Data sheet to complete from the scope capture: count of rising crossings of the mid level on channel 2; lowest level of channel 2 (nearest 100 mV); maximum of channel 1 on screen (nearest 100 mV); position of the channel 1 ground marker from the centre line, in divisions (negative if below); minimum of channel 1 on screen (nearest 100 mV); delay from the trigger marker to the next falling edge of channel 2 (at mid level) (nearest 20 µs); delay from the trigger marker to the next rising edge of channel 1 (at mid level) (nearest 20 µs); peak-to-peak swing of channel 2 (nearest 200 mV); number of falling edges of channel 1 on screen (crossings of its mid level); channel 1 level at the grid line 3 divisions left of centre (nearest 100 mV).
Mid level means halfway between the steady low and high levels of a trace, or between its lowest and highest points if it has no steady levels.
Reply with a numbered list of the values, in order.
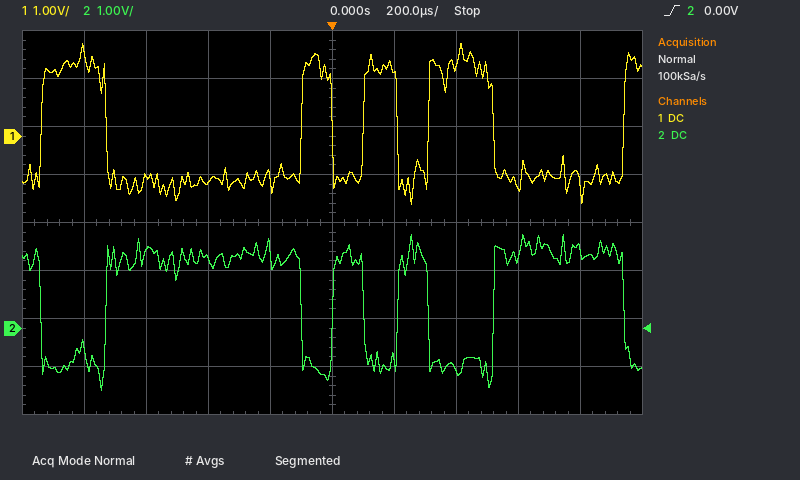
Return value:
1. 4
2. -1.3 V
3. 1.9 V
4. +1.8 div
5. -1.4 V
6. 100 µs
7. 100 µs
8. 3.2 V
9. 4
10. -900 mV
